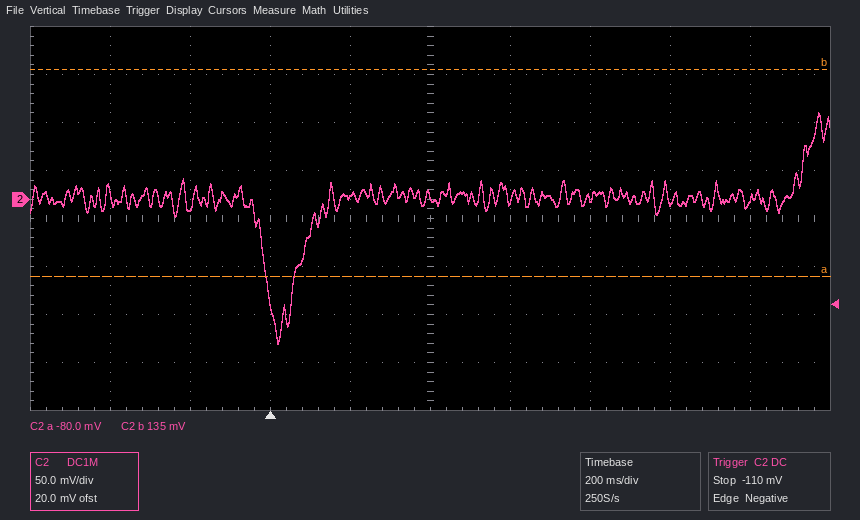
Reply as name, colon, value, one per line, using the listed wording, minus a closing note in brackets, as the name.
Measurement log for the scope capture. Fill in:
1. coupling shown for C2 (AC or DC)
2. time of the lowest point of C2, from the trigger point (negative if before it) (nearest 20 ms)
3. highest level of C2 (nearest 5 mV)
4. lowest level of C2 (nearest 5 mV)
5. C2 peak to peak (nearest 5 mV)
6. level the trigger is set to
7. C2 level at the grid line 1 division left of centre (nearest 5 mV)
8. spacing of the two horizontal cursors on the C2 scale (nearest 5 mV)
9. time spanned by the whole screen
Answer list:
coupling shown for C2: DC
time of the lowest point of C2, from the trigger point (negative if before it): +20 ms
highest level of C2: 90 mV
lowest level of C2: -150 mV
C2 peak to peak: 240 mV
level the trigger is set to: -110 mV
C2 level at the grid line 1 division left of centre: 5 mV
spacing of the two horizontal cursors on the C2 scale: 215 mV
time spanned by the whole screen: 2 s
